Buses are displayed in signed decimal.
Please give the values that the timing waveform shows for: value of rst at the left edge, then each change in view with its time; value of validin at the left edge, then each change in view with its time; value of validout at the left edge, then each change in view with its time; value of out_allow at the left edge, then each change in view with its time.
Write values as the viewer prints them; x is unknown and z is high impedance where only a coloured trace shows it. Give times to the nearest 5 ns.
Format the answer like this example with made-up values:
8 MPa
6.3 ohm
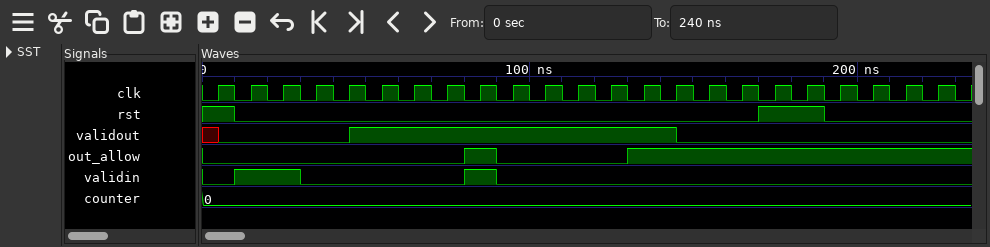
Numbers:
1, 0 at 10 ns, 1 at 170 ns, 0 at 190 ns
0, 1 at 10 ns, 0 at 30 ns, 1 at 80 ns, 0 at 90 ns
x, 0 at 5 ns, 1 at 45 ns, 0 at 145 ns
0, 1 at 80 ns, 0 at 90 ns, 1 at 130 ns
